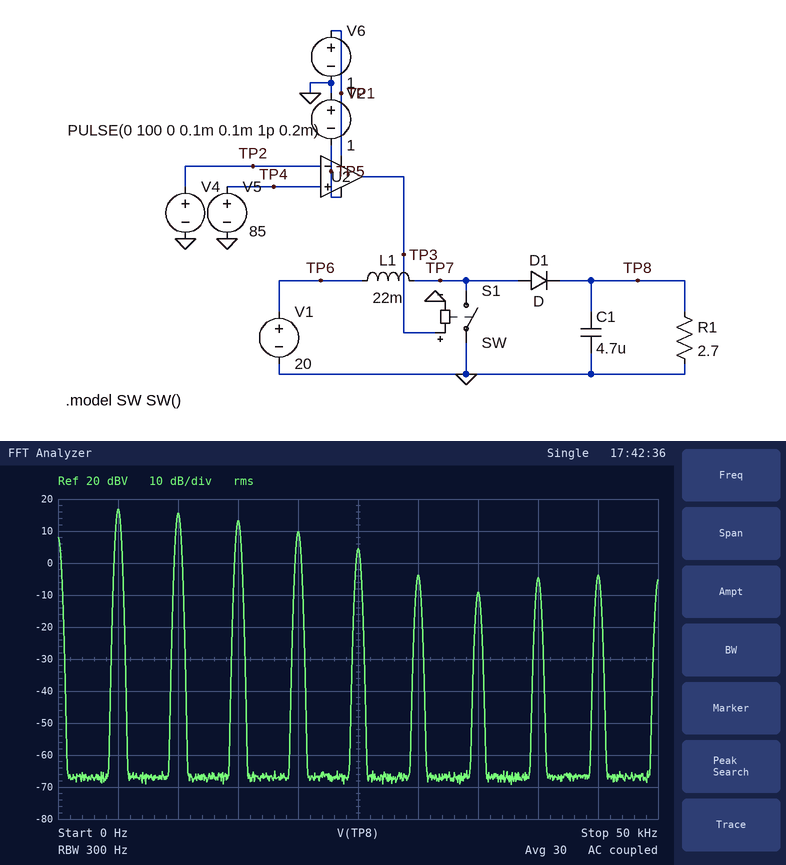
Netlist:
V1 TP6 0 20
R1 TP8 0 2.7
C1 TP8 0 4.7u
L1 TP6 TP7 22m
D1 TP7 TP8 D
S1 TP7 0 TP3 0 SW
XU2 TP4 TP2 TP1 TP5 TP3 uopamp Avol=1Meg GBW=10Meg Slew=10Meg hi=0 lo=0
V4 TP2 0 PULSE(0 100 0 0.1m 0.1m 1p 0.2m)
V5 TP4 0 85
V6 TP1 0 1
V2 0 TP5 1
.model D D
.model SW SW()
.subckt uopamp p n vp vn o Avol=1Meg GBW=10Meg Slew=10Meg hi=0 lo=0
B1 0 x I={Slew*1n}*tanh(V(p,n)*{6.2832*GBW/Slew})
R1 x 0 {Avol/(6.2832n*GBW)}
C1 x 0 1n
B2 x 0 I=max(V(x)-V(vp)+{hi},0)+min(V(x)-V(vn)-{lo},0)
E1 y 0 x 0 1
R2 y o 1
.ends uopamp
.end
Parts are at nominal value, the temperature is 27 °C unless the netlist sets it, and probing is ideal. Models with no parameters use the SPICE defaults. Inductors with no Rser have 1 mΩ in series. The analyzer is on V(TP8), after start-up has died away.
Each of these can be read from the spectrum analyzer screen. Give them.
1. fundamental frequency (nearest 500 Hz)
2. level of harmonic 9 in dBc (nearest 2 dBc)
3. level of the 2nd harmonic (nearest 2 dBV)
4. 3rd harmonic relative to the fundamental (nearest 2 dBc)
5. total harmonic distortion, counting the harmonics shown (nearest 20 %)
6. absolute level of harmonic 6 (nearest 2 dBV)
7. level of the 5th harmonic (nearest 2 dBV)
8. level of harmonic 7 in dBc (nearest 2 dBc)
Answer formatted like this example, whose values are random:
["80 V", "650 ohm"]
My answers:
["5.0 kHz", "-20 dBc", "16 dBV", "-4 dBc", "120 %", "-4 dBV", "4 dBV", "-26 dBc"]
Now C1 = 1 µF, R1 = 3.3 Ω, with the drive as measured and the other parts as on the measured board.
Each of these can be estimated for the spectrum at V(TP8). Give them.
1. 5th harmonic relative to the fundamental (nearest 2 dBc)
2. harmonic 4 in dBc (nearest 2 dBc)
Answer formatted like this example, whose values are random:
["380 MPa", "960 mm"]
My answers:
["-10 dBc", "-6 dBc"]
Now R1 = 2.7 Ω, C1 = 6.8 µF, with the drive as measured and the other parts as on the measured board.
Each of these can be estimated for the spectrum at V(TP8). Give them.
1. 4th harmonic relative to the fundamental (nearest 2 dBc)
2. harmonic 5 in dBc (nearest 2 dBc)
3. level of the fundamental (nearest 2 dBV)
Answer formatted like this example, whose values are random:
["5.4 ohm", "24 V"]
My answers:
["-8 dBc", "-14 dBc", "16 dBV"]
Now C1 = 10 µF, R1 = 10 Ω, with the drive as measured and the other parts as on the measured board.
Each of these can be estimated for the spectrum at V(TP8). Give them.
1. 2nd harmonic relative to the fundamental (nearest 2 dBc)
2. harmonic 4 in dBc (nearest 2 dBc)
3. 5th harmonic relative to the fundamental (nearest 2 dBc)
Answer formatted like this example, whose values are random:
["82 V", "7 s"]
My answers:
["-8 dBc", "-18 dBc", "-24 dBc"]
